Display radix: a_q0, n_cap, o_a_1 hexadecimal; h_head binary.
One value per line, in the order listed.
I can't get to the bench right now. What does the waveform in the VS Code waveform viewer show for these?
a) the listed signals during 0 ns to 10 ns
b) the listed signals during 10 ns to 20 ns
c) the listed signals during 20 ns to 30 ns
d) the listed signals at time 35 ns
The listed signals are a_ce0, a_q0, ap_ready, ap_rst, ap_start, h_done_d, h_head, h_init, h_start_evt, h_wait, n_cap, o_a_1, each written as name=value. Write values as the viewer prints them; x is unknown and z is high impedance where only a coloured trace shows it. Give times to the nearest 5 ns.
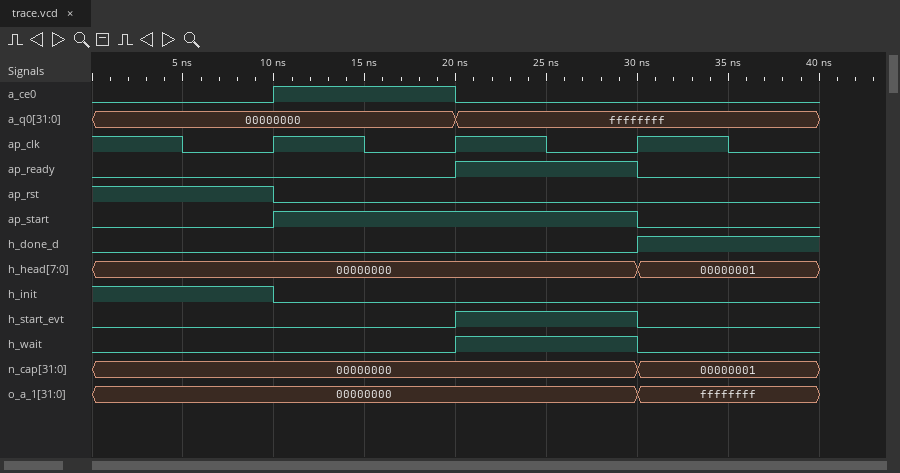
a_ce0=0, a_q0=00000000, ap_ready=0, ap_rst=1, ap_start=0, h_done_d=0, h_head=00000000, h_init=1, h_start_evt=0, h_wait=0, n_cap=00000000, o_a_1=00000000
a_ce0=1, a_q0=00000000, ap_ready=0, ap_rst=0, ap_start=1, h_done_d=0, h_head=00000000, h_init=0, h_start_evt=0, h_wait=0, n_cap=00000000, o_a_1=00000000
a_ce0=0, a_q0=ffffffff, ap_ready=1, ap_rst=0, ap_start=1, h_done_d=0, h_head=00000000, h_init=0, h_start_evt=1, h_wait=1, n_cap=00000000, o_a_1=00000000
a_ce0=0, a_q0=ffffffff, ap_ready=0, ap_rst=0, ap_start=0, h_done_d=1, h_head=00000001, h_init=0, h_start_evt=0, h_wait=0, n_cap=00000001, o_a_1=ffffffff
